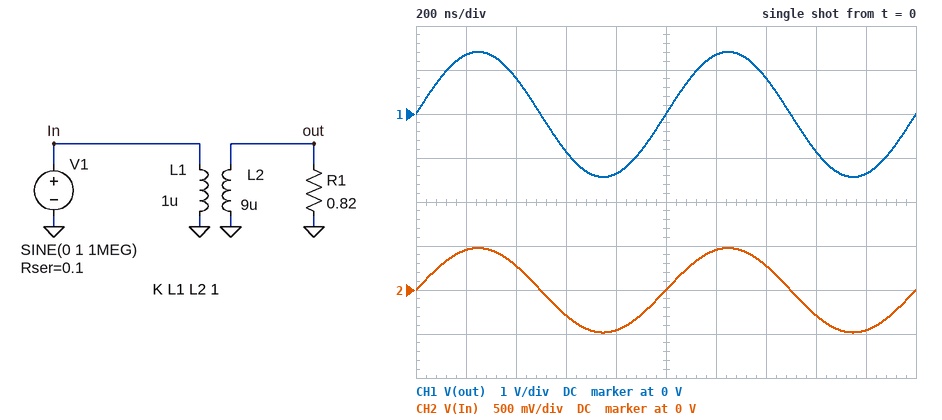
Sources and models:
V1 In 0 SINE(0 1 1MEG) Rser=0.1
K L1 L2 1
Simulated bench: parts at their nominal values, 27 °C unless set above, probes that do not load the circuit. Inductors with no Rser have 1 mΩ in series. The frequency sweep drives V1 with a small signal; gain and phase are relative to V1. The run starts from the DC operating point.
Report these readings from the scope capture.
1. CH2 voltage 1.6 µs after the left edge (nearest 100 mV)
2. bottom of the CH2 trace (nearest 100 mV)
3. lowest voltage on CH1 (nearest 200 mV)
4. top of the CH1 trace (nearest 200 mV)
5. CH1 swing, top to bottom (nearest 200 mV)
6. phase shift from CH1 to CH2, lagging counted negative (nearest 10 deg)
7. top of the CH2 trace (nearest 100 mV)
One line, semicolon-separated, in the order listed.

-300 mV; -500 mV; -1.4 V; 1.4 V; 2.8 V; 0 deg; 500 mV
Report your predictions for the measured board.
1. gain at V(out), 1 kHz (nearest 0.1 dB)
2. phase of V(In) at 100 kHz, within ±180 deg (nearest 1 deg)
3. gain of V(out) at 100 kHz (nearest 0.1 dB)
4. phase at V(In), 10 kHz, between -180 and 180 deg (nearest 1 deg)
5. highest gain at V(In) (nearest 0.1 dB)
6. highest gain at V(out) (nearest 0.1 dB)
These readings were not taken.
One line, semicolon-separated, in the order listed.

-14.7 dB; 4 deg; 3.0 dB; 36 deg; -6.4 dB; 3.1 dB
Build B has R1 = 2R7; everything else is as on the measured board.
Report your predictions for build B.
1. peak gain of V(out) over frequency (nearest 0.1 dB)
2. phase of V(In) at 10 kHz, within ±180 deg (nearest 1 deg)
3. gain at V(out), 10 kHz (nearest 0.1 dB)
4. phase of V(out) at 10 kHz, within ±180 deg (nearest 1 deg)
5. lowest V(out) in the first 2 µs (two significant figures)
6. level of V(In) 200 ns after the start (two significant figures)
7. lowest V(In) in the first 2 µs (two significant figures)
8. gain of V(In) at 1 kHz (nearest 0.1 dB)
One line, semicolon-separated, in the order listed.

7.0 dB; 49 deg; 3.1 dB; 50 deg; -2.3 V; 710 mV; -760 mV; -24.0 dB
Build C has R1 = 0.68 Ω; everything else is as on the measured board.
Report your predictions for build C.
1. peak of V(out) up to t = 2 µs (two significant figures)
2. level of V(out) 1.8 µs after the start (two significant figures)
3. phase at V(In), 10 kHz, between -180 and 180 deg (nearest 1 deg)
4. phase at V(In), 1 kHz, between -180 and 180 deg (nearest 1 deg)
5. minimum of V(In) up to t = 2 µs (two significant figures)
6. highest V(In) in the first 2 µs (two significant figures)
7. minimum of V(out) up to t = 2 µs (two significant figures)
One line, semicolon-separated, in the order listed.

1.3 V; -1.2 V; 34 deg; 73 deg; -440 mV; 430 mV; -1.3 V
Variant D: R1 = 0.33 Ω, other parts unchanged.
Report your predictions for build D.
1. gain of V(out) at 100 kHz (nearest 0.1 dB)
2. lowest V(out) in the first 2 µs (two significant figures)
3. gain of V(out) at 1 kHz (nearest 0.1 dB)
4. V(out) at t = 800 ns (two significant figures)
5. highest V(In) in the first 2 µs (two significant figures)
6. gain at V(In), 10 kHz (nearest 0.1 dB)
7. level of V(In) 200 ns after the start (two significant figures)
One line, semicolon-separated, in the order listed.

-2.0 dB; -800 mV; -14.8 dB; -760 mV; 270 mV; -12.0 dB; 260 mV
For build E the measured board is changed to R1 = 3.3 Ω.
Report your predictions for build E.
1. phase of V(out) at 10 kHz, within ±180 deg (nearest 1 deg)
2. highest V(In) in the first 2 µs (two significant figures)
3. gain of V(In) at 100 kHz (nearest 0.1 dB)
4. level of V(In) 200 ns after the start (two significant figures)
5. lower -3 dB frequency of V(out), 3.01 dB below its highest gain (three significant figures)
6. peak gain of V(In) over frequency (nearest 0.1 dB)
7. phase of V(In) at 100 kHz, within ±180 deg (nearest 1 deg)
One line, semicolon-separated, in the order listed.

52 deg; 780 mV; -2.2 dB; 740 mV; 12.6 kHz; -2.1 dB; 7 deg
